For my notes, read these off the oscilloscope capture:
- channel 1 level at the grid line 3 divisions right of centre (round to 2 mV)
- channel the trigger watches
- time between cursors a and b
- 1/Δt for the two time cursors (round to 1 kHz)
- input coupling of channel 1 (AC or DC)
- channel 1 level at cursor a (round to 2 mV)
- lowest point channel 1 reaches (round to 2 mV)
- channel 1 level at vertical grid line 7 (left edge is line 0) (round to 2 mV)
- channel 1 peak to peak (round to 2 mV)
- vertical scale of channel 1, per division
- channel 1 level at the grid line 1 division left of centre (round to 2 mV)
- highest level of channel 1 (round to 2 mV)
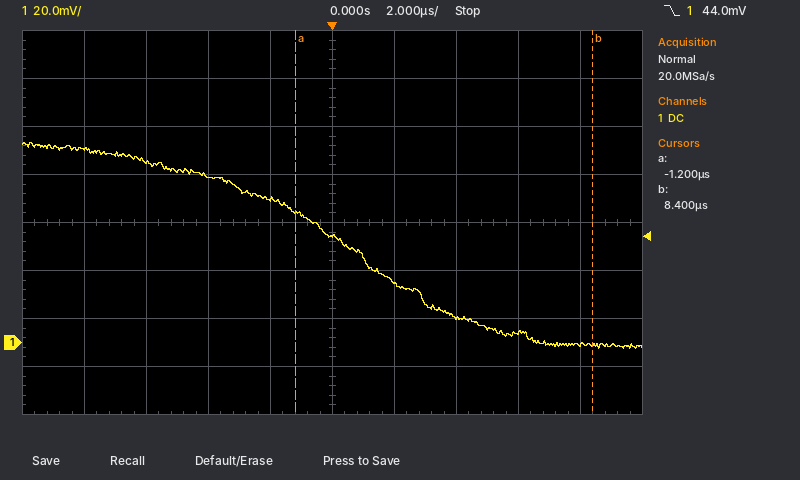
4 mV
channel 1
9.6 µs
104 kHz
DC
54 mV
-2 mV
10 mV
86 mV
20 mV
60 mV
84 mV
